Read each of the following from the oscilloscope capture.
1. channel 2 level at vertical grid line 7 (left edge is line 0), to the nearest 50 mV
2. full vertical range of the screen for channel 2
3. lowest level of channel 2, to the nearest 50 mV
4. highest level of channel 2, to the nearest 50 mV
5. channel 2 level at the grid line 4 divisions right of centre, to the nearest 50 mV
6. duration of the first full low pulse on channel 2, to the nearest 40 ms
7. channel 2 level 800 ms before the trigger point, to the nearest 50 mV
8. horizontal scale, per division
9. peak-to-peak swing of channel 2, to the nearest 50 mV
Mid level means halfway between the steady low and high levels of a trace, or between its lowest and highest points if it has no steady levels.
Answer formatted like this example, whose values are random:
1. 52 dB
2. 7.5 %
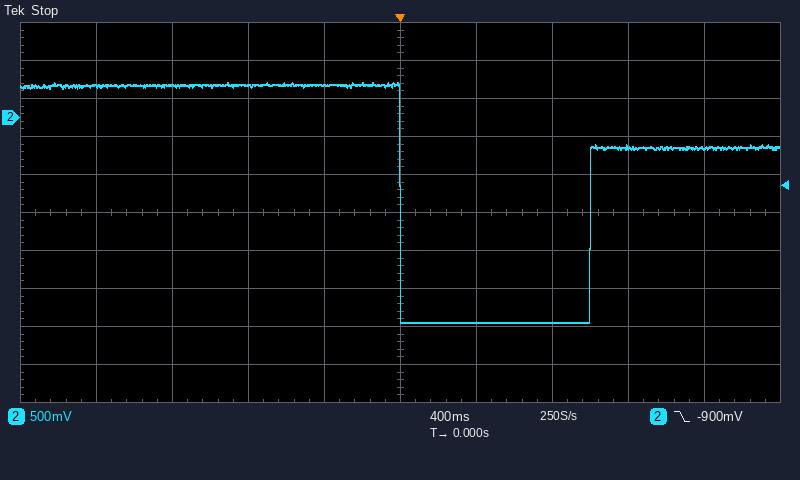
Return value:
1. -2.70 V
2. 5 V
3. -2.70 V
4. 450 mV
5. -400 mV
6. 1.00 s
7. 400 mV
8. 400 ms
9. 3.15 V
